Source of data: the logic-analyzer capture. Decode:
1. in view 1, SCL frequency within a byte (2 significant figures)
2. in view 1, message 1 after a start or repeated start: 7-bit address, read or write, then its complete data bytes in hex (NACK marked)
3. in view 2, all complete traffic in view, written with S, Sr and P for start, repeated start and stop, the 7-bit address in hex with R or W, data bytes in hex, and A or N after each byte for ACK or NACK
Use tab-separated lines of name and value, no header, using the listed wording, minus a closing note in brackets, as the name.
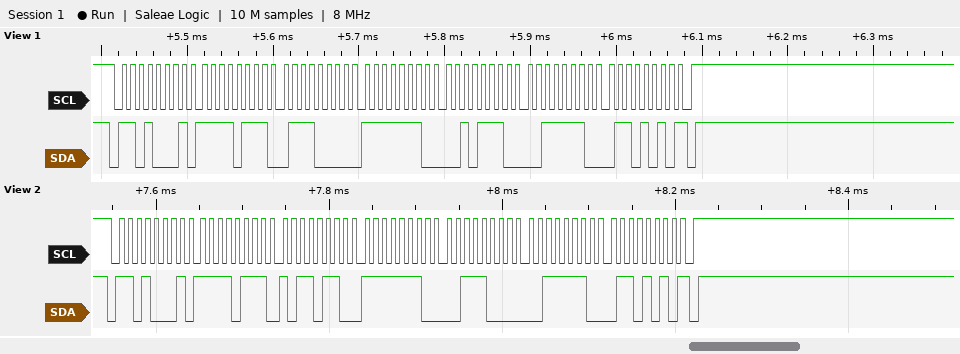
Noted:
in view 1, SCL frequency within a byte	100 kHz
in view 1, message 1 after a start or repeated start: 7-bit address, read or write, then its complete data bytes in hex	0x68 read: F7 70 FE 2E 3E 6A NACK
in view 2, all complete traffic in view, written with S, Sr and P for start, repeated start and stop, the 7-bit address in hex with R or W, data bytes in hex, and A or N after each byte for ACK or NACK	S 68R A F7 A B6 A FE A 38 A 3E A 6A N P
